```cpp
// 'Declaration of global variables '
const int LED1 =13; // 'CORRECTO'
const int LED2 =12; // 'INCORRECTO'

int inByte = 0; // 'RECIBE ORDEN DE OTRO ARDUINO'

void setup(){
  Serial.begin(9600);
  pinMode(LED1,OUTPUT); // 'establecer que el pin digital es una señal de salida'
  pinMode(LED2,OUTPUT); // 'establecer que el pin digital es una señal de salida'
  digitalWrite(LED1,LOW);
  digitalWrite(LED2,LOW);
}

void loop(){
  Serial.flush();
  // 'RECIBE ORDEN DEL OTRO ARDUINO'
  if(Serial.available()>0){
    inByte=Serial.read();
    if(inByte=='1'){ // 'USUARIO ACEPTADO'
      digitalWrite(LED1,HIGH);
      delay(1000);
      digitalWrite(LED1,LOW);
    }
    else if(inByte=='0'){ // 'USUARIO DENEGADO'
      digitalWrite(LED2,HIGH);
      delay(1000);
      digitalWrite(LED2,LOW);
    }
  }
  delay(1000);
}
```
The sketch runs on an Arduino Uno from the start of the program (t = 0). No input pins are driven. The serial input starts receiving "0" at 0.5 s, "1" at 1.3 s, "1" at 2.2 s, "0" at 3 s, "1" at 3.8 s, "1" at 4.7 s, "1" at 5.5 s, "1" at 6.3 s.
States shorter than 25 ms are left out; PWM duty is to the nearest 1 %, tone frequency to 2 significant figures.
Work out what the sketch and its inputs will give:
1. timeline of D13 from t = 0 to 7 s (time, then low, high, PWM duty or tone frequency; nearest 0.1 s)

0 s low; 3 s high; 4 s low; 5 s high; 6 s low
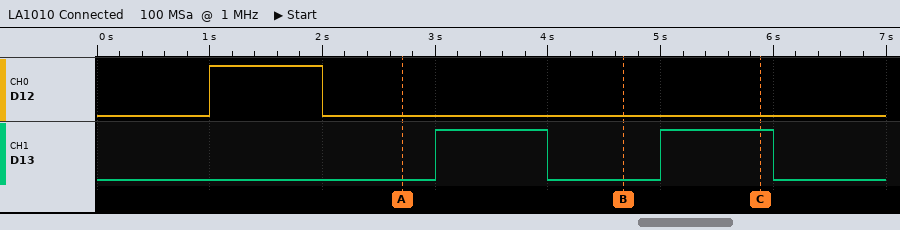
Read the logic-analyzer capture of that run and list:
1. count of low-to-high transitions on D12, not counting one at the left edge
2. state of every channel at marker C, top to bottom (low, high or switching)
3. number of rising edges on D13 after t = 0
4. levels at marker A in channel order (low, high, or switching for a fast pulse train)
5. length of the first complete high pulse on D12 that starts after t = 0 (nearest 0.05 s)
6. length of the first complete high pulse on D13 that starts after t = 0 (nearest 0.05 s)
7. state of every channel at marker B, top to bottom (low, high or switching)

1
D12 low, D13 high
2
D12 low, D13 low
1.00 s
1.00 s
D12 low, D13 low
